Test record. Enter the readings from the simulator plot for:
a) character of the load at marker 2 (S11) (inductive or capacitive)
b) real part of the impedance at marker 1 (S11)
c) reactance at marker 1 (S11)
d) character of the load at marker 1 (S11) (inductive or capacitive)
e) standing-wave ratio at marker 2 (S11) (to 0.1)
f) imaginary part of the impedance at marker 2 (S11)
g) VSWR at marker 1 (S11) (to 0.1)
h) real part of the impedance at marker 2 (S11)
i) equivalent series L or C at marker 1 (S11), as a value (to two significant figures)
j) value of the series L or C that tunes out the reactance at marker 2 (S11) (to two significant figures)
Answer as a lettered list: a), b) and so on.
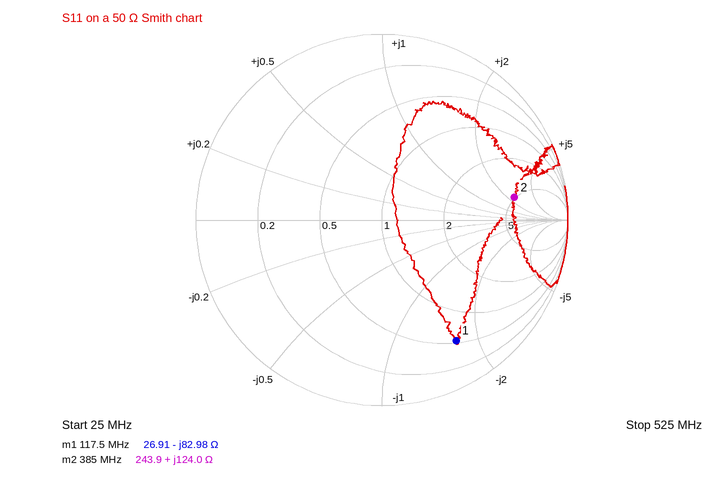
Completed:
a) inductive
b) 26.91 Ω
c) -82.98 Ω
d) capacitive
e) 6.2
f) +124.0 Ω
g) 7.4
h) 243.9 Ω
i) 16 pF
j) 3.3 pF
